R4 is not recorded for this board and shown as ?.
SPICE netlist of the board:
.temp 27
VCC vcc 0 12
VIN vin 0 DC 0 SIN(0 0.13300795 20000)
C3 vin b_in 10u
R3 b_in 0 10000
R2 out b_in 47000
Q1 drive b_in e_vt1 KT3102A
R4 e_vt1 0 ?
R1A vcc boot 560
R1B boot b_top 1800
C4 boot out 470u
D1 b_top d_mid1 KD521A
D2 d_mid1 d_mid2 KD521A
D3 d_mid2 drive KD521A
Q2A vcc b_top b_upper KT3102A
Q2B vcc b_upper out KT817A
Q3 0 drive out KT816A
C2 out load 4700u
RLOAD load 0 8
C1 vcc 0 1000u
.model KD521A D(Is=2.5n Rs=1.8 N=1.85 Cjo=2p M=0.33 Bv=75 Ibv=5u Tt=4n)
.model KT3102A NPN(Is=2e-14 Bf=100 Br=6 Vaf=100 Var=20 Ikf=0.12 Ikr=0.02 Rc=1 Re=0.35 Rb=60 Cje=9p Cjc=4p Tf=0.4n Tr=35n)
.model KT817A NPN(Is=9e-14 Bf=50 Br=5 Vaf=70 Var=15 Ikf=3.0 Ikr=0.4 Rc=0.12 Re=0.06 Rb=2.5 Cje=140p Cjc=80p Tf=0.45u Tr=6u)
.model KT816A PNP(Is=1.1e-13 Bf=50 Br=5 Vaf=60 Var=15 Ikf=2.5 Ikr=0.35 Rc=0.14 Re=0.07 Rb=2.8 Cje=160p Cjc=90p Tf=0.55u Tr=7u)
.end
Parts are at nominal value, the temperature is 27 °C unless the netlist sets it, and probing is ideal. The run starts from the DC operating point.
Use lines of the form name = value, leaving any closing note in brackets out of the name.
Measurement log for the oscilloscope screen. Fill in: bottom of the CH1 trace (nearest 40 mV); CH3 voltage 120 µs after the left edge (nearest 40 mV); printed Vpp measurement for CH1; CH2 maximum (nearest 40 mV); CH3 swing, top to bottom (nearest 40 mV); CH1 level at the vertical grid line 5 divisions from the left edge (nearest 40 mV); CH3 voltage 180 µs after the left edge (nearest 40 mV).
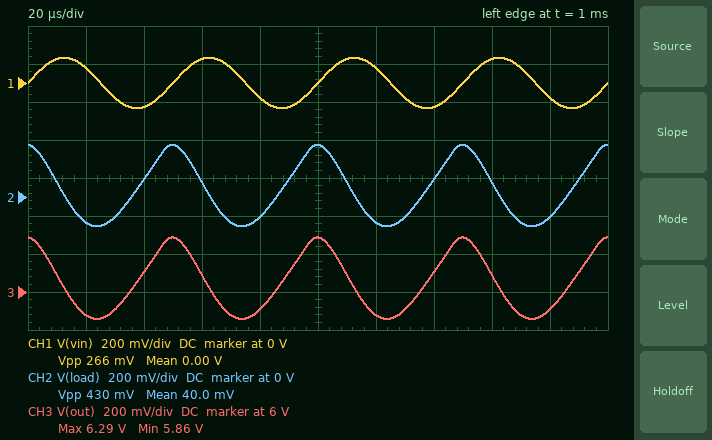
bottom of the CH1 trace = -120 mV
CH3 voltage 120 µs after the left edge = 5.88 V
printed Vpp measurement for CH1 = 266 mV
CH2 maximum = 280 mV
CH3 swing, top to bottom = 440 mV
CH1 level at the vertical grid line 5 divisions from the left edge = 0 V
CH3 voltage 180 µs after the left edge = 5.92 V
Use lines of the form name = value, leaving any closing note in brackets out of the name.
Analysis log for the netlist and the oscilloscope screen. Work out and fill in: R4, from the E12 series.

R4, from the E12 series = 82 Ω
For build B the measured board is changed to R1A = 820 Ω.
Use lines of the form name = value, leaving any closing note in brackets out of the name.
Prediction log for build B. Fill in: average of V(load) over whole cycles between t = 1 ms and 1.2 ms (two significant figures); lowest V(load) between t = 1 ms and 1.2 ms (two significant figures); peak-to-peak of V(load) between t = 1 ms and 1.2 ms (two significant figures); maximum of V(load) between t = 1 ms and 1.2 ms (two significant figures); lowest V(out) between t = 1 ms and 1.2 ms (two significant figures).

average of V(load) over whole cycles between t = 1 ms and 1.2 ms = 72 mV
lowest V(load) between t = 1 ms and 1.2 ms = -130 mV
peak-to-peak of V(load) between t = 1 ms and 1.2 ms = 490 mV
maximum of V(load) between t = 1 ms and 1.2 ms = 360 mV
lowest V(out) between t = 1 ms and 1.2 ms = 5.7 V
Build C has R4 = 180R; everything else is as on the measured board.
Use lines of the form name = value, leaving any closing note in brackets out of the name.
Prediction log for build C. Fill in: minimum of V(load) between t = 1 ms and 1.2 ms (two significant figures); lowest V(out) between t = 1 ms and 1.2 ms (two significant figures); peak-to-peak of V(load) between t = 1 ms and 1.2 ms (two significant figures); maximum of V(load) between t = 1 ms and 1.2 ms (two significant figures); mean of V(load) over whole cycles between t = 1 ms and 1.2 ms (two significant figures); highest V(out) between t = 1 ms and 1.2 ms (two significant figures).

minimum of V(load) between t = 1 ms and 1.2 ms = -81 mV
lowest V(out) between t = 1 ms and 1.2 ms = 6.6 V
peak-to-peak of V(load) between t = 1 ms and 1.2 ms = 190 mV
maximum of V(load) between t = 1 ms and 1.2 ms = 110 mV
mean of V(load) over whole cycles between t = 1 ms and 1.2 ms = 9.5 mV
highest V(out) between t = 1 ms and 1.2 ms = 6.8 V
